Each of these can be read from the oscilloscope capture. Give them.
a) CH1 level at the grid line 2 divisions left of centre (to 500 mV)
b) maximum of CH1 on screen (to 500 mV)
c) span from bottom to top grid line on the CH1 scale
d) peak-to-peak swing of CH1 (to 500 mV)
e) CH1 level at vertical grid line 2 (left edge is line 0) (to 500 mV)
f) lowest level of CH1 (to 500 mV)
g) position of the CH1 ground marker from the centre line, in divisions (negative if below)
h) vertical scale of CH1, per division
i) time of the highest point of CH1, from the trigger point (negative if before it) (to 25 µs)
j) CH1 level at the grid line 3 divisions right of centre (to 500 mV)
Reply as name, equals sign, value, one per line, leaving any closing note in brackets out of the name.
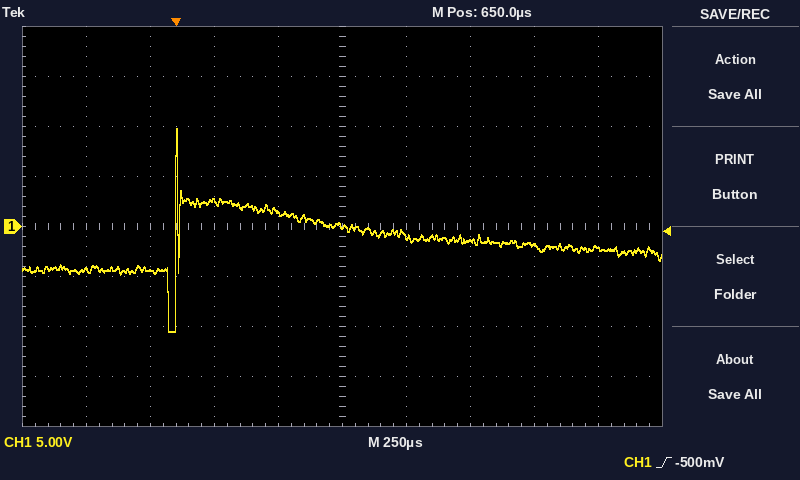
CH1 level at the grid line 2 divisions left of centre = 2.5 V
maximum of CH1 on screen = 10.0 V
span from bottom to top grid line on the CH1 scale = 40 V
peak-to-peak swing of CH1 = 20.5 V
CH1 level at vertical grid line 2 (left edge is line 0) = -4.5 V
lowest level of CH1 = -10.5 V
position of the CH1 ground marker from the centre line, in divisions = 0.0 div
vertical scale of CH1, per division = 5 V
time of the highest point of CH1, from the trigger point (negative if before it) = 0 µs
CH1 level at the grid line 3 divisions right of centre = -2.0 V
